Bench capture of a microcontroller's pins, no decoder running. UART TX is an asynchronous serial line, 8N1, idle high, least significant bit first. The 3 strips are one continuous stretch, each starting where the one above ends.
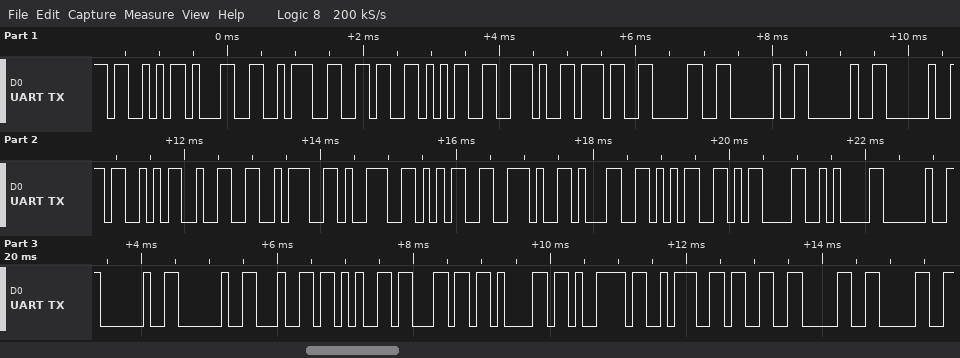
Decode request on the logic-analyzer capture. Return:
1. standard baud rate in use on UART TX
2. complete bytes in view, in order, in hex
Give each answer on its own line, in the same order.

9600 baud
53 31 3A 36 35 2E 37 30 20 20 20 53 32 3A 39 35 2E 31 35 0D 0A 20 20 20 64 65 6C 61 79 3A 33 30 30
